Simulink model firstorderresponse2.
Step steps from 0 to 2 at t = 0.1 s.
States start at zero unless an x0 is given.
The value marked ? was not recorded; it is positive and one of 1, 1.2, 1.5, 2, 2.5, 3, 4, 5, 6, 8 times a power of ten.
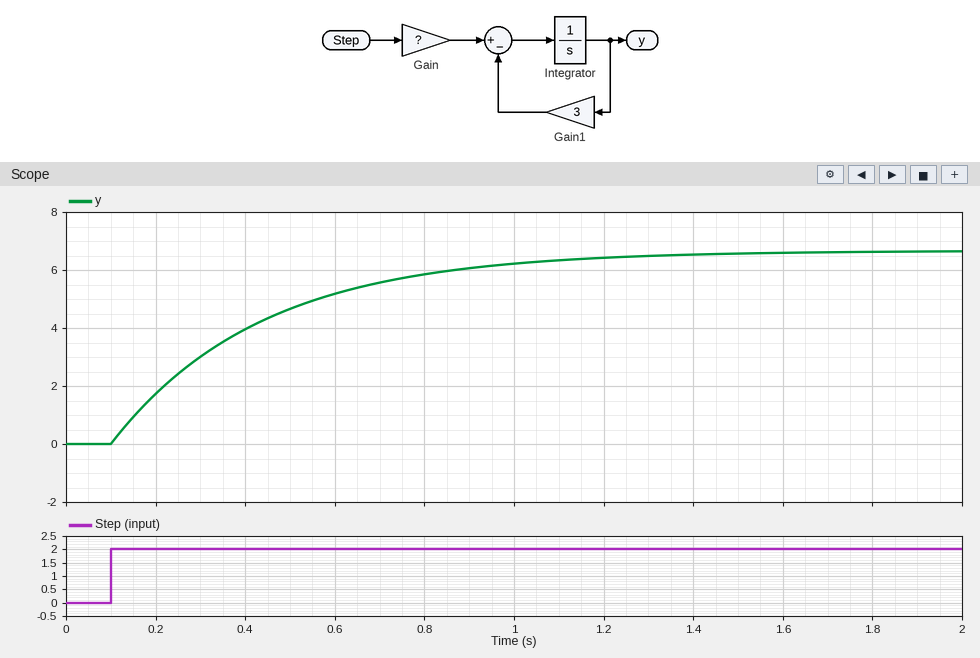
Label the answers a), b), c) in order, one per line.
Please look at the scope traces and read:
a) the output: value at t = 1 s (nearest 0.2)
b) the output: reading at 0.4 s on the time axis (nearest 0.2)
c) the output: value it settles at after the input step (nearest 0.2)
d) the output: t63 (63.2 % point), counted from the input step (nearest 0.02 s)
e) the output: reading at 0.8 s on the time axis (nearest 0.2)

a) 6.2
b) 4.0
c) 6.6
d) 0.34 s
e) 5.8
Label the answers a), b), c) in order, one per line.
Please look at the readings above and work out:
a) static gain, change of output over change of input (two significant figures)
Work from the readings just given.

a) 3.3
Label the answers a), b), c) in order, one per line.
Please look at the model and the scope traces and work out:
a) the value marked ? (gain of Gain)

a) 10
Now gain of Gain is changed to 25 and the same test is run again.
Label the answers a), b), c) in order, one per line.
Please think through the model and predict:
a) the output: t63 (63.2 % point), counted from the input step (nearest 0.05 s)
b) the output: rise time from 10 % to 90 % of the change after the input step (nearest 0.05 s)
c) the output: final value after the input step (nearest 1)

a) 0.35 s
b) 0.75 s
c) 17
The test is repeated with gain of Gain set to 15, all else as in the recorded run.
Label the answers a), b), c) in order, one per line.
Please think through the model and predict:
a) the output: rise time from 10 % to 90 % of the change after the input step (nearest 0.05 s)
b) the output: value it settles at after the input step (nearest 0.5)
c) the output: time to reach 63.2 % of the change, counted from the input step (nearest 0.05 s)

a) 0.75 s
b) 10.0
c) 0.35 s
